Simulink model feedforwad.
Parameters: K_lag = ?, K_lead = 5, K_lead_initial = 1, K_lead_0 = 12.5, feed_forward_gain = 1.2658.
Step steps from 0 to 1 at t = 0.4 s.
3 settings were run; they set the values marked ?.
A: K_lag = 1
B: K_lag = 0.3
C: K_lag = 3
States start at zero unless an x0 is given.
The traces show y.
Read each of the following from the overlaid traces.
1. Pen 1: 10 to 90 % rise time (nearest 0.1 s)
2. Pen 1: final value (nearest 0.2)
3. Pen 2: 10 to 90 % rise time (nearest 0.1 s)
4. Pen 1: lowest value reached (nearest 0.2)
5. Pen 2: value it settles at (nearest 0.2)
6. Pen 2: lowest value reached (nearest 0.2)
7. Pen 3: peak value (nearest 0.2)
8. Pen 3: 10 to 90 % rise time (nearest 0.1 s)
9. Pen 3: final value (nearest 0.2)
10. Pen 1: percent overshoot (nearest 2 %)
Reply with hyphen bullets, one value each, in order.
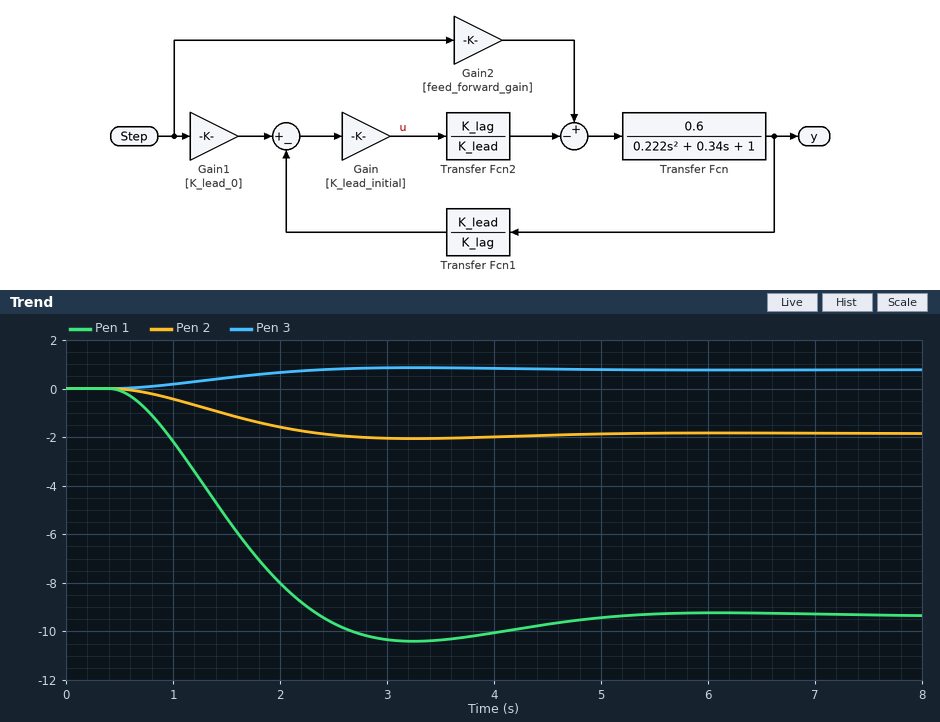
- 1.3 s
- -9.4
- 1.3 s
- -10.4
- -1.8
- -2.0
- 0.8
- 1.3 s
- 0.8
- 12 %
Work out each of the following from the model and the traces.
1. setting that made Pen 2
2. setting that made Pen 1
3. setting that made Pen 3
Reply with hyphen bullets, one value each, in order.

- A
- C
- B
